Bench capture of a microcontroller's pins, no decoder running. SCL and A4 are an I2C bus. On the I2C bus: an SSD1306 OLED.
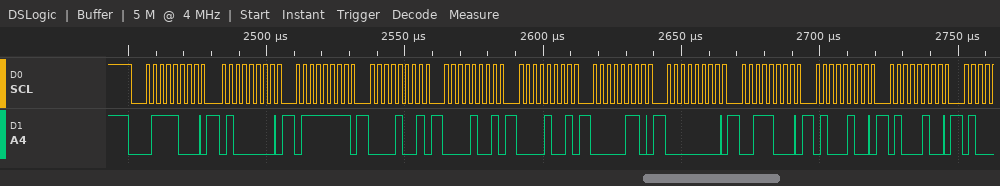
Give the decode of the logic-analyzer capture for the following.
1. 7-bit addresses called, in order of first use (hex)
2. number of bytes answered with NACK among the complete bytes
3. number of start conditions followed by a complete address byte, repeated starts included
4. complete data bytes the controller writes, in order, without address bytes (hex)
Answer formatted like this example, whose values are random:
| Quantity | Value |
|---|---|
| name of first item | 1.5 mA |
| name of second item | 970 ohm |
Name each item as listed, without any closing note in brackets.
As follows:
| Quantity | Value |
|---|---|
| 7-bit addresses called, in order of first use | 0x3C |
| number of bytes answered with NACK among the complete bytes | 0 |
| number of start conditions followed by a complete address byte, repeated starts included | 1 |
| complete data bytes the controller writes, in order, without address bytes | 40 7F 09 09 09 06 00 38 44 44 |
